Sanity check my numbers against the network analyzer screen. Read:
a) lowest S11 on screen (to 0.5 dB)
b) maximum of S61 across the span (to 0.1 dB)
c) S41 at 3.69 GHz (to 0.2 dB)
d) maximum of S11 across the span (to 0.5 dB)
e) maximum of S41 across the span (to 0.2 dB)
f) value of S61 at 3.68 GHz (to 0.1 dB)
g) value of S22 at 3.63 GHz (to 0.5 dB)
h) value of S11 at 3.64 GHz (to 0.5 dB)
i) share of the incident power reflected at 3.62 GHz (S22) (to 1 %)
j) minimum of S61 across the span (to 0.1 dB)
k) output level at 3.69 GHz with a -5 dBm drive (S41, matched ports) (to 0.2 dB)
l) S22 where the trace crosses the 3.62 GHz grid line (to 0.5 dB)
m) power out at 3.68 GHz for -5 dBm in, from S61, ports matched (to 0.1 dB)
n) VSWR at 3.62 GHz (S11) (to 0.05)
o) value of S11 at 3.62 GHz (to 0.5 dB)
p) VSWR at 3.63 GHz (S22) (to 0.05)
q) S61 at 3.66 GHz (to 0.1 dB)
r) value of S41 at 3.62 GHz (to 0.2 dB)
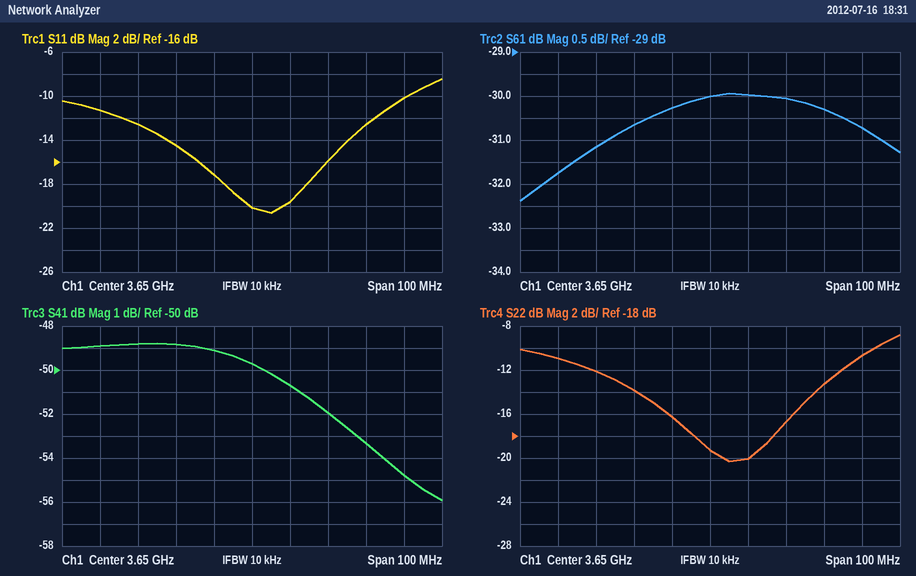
-20.5 dB
-29.9 dB
-54.8 dB
-8.5 dB
-48.8 dB
-30.3 dB
-14.0 dB
-17.0 dB
6 %
-32.4 dB
-59.8 dBm
-12.0 dB
-35.3 dBm
1.60
-12.5 dB
1.50
-30.0 dB
-48.8 dB
